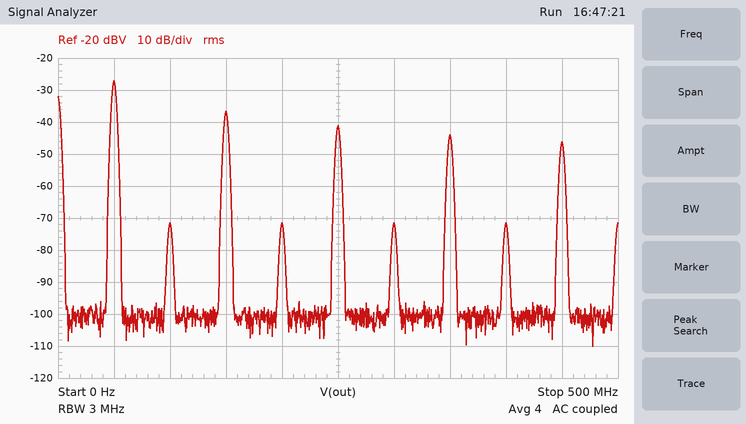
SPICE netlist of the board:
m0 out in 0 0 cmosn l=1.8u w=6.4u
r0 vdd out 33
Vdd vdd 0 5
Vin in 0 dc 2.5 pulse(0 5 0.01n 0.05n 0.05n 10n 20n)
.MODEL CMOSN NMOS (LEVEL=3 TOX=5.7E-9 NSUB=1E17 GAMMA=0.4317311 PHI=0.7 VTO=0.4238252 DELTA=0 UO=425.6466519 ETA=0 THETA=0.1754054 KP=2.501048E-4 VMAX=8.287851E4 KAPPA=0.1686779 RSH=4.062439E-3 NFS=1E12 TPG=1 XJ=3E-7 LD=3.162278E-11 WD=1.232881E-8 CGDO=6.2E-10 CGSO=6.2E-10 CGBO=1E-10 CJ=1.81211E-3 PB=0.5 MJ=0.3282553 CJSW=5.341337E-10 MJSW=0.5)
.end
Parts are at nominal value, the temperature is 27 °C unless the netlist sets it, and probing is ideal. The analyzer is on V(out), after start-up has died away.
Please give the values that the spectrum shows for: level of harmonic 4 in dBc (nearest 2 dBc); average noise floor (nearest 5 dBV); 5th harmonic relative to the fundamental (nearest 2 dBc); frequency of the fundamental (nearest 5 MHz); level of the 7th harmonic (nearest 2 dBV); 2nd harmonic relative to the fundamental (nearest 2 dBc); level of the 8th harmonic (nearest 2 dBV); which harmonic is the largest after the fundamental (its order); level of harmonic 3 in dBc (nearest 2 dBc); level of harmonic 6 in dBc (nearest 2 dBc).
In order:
-44 dBc
-100 dBV
-14 dBc
50 MHz
-44 dBV
-44 dBc
-72 dBV
3
-10 dBc
-44 dBc
